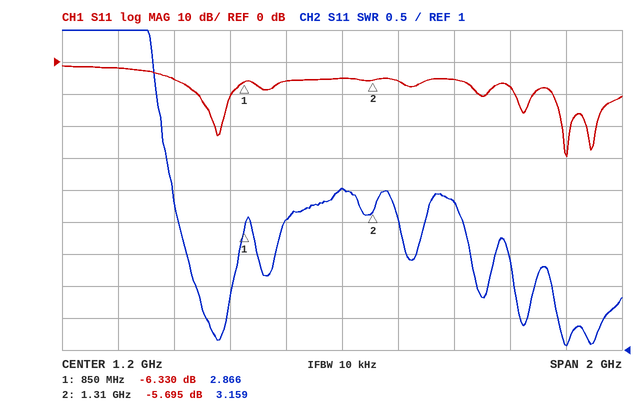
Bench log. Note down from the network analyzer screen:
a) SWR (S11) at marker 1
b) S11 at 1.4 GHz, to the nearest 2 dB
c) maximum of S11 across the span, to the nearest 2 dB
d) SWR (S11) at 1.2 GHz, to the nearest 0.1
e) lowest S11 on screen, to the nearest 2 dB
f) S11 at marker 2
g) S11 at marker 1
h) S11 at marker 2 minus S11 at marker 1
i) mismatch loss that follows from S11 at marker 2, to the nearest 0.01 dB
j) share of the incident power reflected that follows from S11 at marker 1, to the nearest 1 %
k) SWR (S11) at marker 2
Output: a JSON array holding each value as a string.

["2.866", "-6 dB", "-2 dB", "3.5", "-30 dB", "-5.695 dB", "-6.330 dB", "0.635 dB", "1.36 dB", "23 %", "3.159"]
